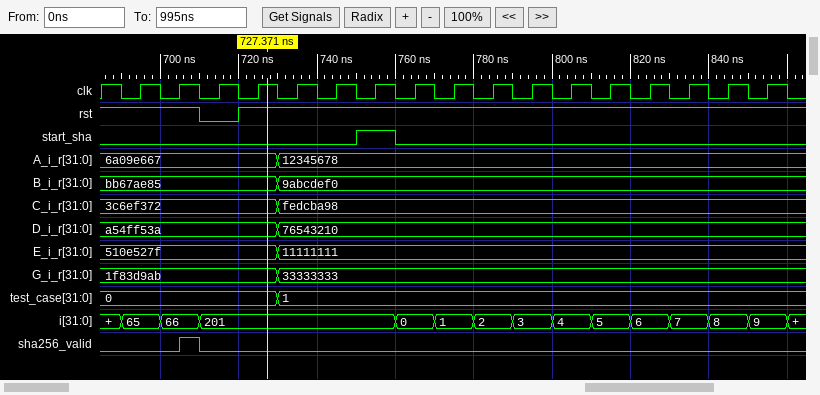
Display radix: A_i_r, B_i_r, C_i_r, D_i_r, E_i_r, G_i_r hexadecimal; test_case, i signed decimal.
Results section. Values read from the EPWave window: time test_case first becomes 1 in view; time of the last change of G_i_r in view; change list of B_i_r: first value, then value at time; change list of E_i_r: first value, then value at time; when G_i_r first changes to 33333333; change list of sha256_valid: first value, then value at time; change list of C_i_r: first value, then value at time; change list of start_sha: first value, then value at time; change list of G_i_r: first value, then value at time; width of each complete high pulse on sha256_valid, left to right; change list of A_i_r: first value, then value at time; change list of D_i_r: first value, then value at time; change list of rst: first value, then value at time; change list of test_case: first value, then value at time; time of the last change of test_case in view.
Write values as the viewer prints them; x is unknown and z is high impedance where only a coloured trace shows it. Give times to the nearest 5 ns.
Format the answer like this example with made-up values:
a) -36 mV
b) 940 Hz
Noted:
a) 730 ns
b) 730 ns
c) bb67ae85, 9abcdef0 at 730 ns
d) 510e527f, 11111111 at 730 ns
e) 730 ns
f) 0, 1 at 705 ns, 0 at 710 ns
g) 3c6ef372, fedcba98 at 730 ns
h) 0, 1 at 750 ns, 0 at 760 ns
i) 1f83d9ab, 33333333 at 730 ns
j) 5 ns
k) 6a09e667, 12345678 at 730 ns
l) a54ff53a, 76543210 at 730 ns
m) 1, 0 at 710 ns, 1 at 720 ns
n) 0, 1 at 730 ns
o) 730 ns
